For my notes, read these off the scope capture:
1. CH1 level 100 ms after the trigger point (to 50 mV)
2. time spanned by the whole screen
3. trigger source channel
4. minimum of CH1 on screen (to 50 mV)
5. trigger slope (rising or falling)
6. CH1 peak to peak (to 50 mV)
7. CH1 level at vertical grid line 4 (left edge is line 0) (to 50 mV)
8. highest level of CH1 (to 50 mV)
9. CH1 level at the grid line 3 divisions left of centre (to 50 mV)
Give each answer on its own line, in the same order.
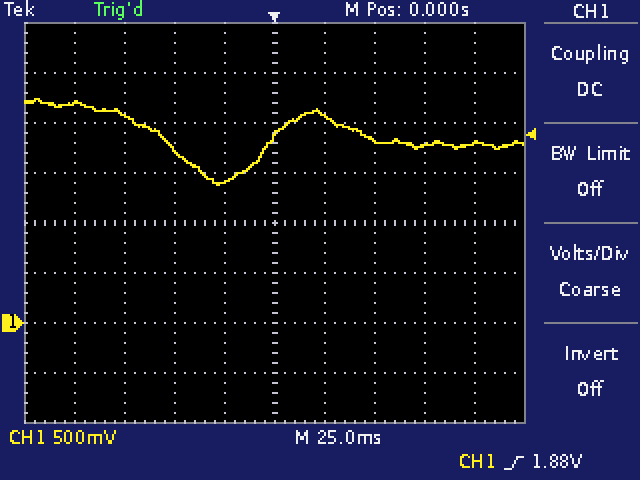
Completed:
1.80 V
250 ms
CH1
1.40 V
rising
850 mV
1.40 V
2.25 V
2.10 V
